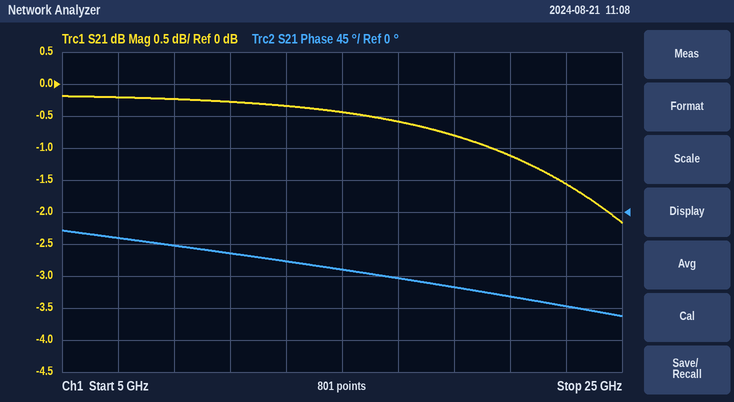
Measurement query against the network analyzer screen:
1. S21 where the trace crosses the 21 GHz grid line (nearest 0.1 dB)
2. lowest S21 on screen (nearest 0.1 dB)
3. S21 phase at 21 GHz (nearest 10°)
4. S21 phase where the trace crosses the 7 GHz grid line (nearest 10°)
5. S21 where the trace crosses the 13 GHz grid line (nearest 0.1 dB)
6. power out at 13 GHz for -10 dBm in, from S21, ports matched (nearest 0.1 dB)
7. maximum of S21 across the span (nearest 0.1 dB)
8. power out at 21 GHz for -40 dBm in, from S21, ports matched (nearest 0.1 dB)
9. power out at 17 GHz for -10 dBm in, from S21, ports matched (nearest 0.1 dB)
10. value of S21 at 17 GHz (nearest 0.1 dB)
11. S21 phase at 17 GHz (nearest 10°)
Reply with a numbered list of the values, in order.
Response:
1. -1.1 dB
2. -2.2 dB
3. -120°
4. -40°
5. -0.3 dB
6. -10.3 dBm
7. -0.2 dB
8. -41.1 dBm
9. -10.6 dBm
10. -0.6 dB
11. -90°
